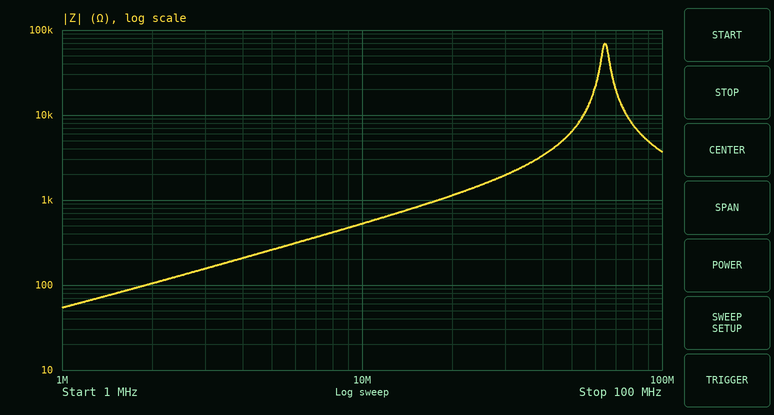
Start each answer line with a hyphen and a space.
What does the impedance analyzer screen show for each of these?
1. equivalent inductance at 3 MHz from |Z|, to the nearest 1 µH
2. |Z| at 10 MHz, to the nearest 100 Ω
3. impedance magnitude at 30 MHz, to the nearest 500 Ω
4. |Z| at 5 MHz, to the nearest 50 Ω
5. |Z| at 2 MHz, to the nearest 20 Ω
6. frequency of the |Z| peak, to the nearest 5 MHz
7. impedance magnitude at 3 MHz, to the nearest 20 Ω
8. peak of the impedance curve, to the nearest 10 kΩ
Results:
- 8 µH
- 500 Ω
- 2.0 kΩ
- 250 Ω
- 100 Ω
- 65 MHz
- 160 Ω
- 70 kΩ
